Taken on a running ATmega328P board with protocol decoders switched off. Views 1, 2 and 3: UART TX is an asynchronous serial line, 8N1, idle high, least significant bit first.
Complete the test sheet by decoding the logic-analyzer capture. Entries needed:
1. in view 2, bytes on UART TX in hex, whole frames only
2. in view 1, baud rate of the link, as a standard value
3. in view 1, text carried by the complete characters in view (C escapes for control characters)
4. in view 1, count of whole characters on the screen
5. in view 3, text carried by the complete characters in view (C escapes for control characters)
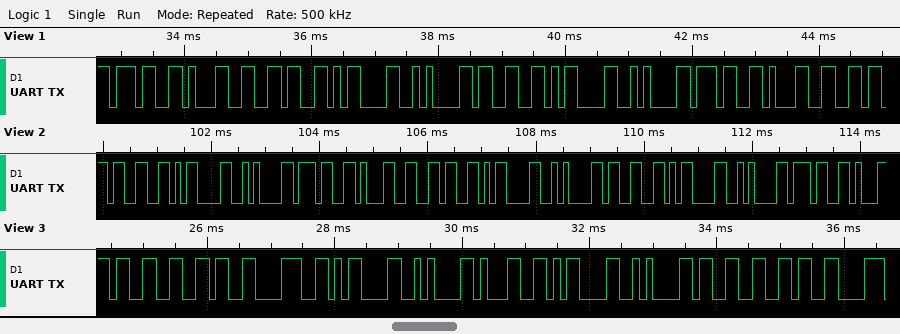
33 0D 0A 37 31 36 0D 0A 33 0D 0A 37
9600 baud
"716\r\n3\r\n71"
10
"368\r\n1\r\n36"
